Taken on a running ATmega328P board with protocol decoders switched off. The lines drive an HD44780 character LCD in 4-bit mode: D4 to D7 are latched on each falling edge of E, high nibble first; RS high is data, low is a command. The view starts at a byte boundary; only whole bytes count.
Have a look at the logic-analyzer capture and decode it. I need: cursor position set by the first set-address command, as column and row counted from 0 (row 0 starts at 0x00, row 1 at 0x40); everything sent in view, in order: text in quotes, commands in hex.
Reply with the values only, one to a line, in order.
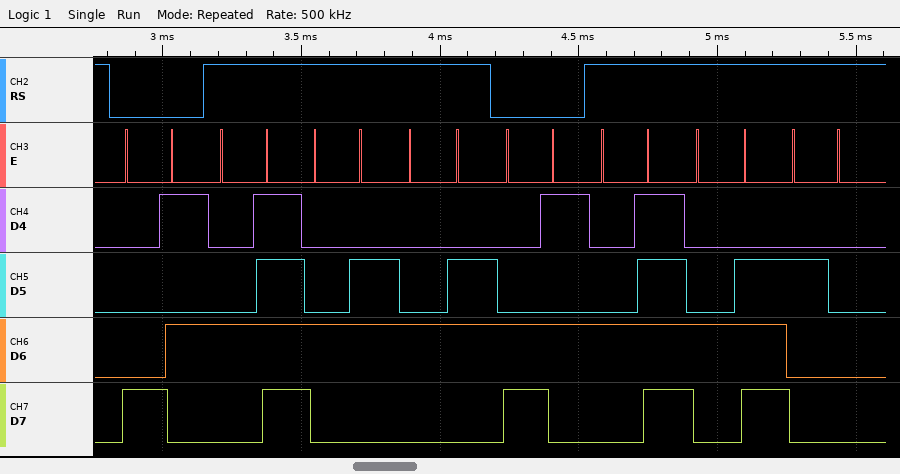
column 5, row 0
0x85 "OFF" 0xC5 "ON "
